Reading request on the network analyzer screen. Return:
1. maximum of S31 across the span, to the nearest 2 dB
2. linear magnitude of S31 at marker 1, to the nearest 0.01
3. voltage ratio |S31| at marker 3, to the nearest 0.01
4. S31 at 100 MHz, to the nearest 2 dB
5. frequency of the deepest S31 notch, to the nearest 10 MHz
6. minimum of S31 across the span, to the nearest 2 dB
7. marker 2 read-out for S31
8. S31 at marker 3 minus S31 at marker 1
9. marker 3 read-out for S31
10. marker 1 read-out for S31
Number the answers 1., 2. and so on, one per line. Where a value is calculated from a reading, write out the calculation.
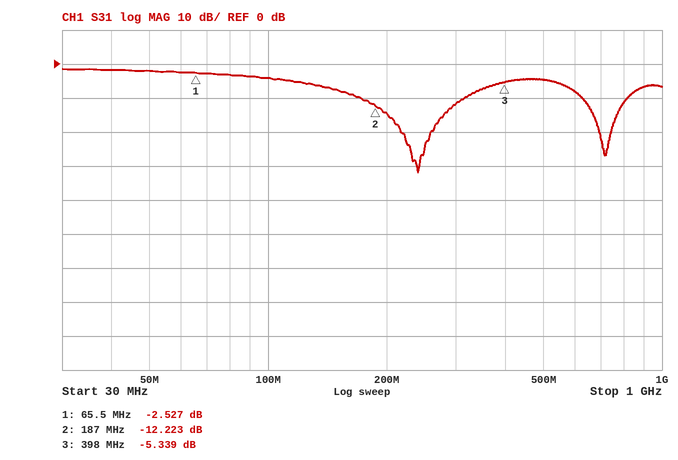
1. -2 dB
2. 10^(-2.527/20) ≈ 0.75
3. 10^(-5.339/20) ≈ 0.54
4. -4 dB
5. 240 MHz
6. -32 dB
7. -12.223 dB
8. -5.339 − (-2.527) = -2.812 dB
9. -5.339 dB
10. -2.527 dB
